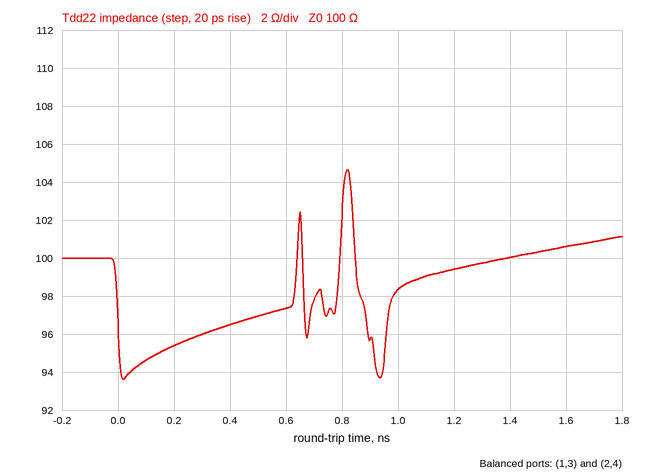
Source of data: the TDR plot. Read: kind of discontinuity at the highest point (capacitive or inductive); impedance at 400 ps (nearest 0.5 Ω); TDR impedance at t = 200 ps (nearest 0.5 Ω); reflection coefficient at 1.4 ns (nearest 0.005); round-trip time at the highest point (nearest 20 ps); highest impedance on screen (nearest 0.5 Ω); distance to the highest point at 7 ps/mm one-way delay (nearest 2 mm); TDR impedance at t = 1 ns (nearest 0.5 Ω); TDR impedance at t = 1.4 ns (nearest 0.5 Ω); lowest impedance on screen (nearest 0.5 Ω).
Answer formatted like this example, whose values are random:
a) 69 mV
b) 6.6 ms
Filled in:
a) inductive
b) 96.5 Ω
c) 95.5 Ω
d) 0.000
e) 820 ps
f) 104.5 Ω
g) 58 mm
h) 98.5 Ω
i) 100.0 Ω
j) 93.5 Ω
